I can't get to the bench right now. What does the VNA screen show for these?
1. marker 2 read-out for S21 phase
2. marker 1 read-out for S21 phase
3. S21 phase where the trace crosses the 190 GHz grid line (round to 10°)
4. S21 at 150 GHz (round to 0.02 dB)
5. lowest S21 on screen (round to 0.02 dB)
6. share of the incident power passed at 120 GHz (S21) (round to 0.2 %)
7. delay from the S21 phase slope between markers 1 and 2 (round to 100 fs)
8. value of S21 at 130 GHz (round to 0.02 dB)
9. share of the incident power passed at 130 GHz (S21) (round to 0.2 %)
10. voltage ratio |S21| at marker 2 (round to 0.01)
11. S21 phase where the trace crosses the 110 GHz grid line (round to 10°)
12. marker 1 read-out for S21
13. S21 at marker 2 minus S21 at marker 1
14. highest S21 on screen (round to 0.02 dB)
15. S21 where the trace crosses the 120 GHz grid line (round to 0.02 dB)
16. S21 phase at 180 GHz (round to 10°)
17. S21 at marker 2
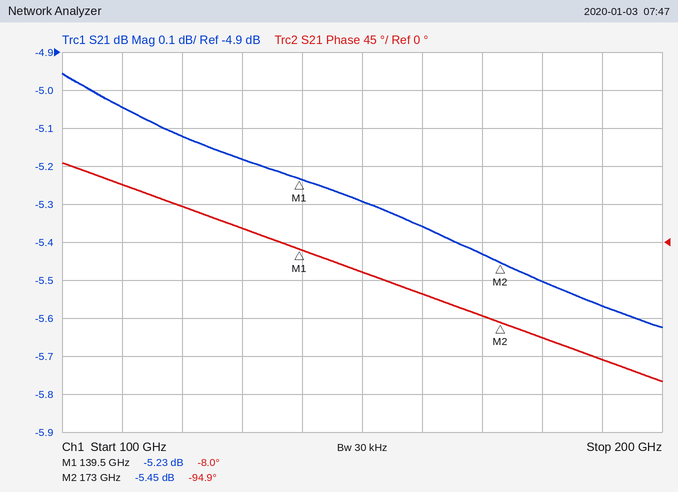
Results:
-94.9°
-8.0°
-140°
-5.30 dB
-5.62 dB
30.8 %
7.2 ps
-5.18 dB
30.4 %
0.53
70°
-5.23 dB
-0.22 dB
-4.96 dB
-5.12 dB
-110°
-5.45 dB
